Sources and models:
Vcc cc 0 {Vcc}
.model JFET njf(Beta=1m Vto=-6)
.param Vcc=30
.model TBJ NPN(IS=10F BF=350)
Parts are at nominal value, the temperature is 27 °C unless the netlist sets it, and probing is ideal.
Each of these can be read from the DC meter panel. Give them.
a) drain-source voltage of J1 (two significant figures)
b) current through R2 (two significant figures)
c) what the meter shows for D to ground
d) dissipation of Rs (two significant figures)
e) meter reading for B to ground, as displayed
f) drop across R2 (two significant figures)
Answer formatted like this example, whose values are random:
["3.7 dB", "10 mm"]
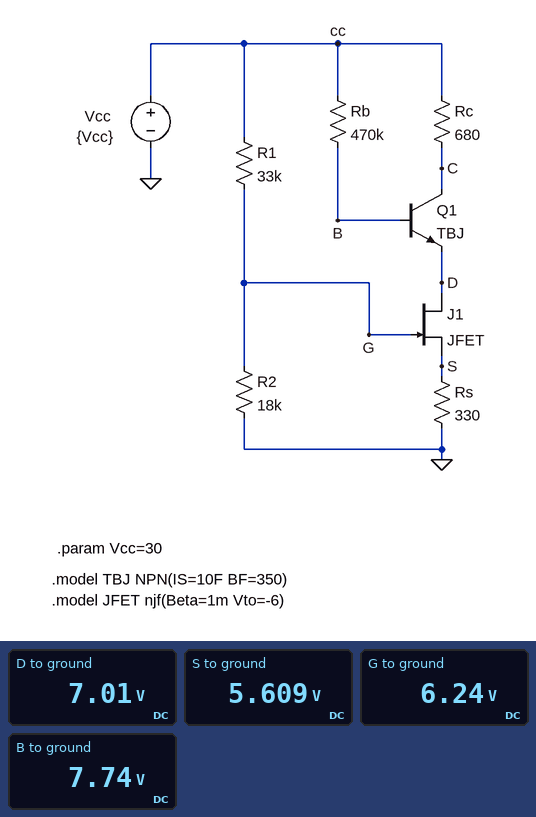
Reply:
["1.4 V", "350 µA", "7.01 V", "95 mW", "7.74 V", "6.2 V"]
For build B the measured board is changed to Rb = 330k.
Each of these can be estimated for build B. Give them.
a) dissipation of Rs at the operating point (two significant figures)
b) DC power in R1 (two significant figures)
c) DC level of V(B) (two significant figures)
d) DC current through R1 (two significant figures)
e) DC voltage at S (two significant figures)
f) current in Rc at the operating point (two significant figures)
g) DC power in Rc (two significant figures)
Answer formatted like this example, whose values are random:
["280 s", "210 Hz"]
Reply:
["160 mW", "15 mW", "9.8 V", "670 µA", "7.2 V", "21 mA", "310 mW"]
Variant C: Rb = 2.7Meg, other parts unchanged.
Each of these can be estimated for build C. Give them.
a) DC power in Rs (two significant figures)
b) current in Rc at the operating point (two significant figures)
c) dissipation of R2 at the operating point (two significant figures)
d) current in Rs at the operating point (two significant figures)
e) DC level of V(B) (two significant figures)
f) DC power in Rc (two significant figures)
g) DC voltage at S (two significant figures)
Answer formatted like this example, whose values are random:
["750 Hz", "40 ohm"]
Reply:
["6.2 mW", "3.6 mA", "240 µW", "4.3 mA", "2.4 V", "8.7 mW", "1.4 V"]
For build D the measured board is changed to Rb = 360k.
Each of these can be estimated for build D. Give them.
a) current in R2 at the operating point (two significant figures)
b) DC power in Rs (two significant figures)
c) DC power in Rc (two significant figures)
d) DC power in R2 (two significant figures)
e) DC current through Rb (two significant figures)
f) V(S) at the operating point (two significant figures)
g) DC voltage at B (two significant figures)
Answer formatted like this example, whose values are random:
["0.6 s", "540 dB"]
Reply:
["410 µA", "140 mW", "280 mW", "3.0 mW", "58 µA", "6.8 V", "9.3 V"]
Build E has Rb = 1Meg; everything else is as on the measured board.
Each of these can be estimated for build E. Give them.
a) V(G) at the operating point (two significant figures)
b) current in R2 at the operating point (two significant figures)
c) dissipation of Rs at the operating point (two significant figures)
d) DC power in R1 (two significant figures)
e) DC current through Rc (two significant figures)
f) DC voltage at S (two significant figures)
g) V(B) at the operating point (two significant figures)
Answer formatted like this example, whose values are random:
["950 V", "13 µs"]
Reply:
["3.8 V", "210 µA", "30 mW", "21 mW", "8.9 mA", "3.1 V", "4.6 V"]
